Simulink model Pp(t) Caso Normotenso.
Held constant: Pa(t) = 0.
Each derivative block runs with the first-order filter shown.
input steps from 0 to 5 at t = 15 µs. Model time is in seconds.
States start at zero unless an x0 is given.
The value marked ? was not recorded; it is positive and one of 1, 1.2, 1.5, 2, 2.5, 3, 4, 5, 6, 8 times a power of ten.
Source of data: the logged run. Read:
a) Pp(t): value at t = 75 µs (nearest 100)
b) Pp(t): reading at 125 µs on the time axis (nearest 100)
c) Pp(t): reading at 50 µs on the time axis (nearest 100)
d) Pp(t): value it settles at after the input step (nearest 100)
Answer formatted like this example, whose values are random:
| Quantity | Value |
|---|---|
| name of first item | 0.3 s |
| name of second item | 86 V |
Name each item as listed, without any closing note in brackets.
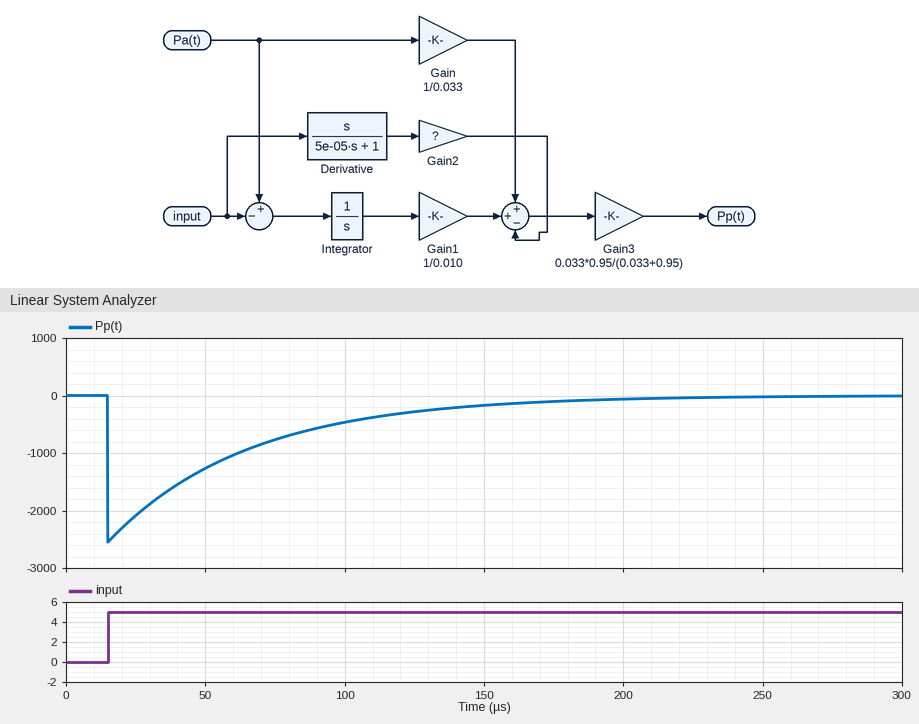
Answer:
| Quantity | Value |
|---|---|
| Pp(t): value at t = 75 µs | -800 |
| Pp(t): reading at 125 µs on the time axis | -300 |
| Pp(t): reading at 50 µs on the time axis | -1300 |
| Pp(t): value it settles at after the input step | 0 |
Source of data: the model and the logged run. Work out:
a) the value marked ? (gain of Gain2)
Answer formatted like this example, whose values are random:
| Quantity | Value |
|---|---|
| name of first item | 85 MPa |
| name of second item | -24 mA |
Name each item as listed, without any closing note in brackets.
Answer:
| Quantity | Value |
|---|---|
| the value marked ? | 0.8 |
